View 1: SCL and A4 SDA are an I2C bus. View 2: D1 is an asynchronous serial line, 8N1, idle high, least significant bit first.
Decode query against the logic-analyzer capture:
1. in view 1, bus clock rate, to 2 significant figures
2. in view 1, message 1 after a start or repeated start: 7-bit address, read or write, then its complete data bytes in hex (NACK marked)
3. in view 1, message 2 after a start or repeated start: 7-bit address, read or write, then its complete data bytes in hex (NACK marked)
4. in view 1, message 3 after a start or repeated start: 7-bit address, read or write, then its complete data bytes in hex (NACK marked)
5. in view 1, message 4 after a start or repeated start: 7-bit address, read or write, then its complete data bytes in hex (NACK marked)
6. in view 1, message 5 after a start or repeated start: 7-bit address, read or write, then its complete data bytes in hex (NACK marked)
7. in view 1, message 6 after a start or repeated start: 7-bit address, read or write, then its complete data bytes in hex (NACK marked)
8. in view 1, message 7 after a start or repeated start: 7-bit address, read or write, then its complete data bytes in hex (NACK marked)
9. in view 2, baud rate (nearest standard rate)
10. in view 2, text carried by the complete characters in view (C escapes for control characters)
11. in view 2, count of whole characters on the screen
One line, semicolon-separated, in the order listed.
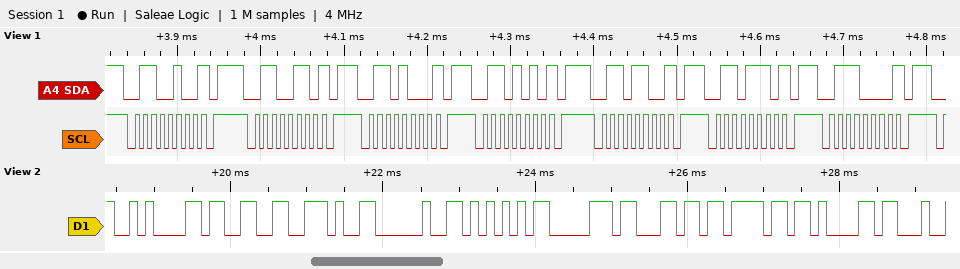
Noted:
100 kHz; 0x32 write NACK; 0x33 write NACK; 0x34 write NACK; 0x35 write NACK; 0x36 write NACK; 0x37 write NACK; 0x38 write NACK; 9600 baud; "\n3. Uploa"; 9
